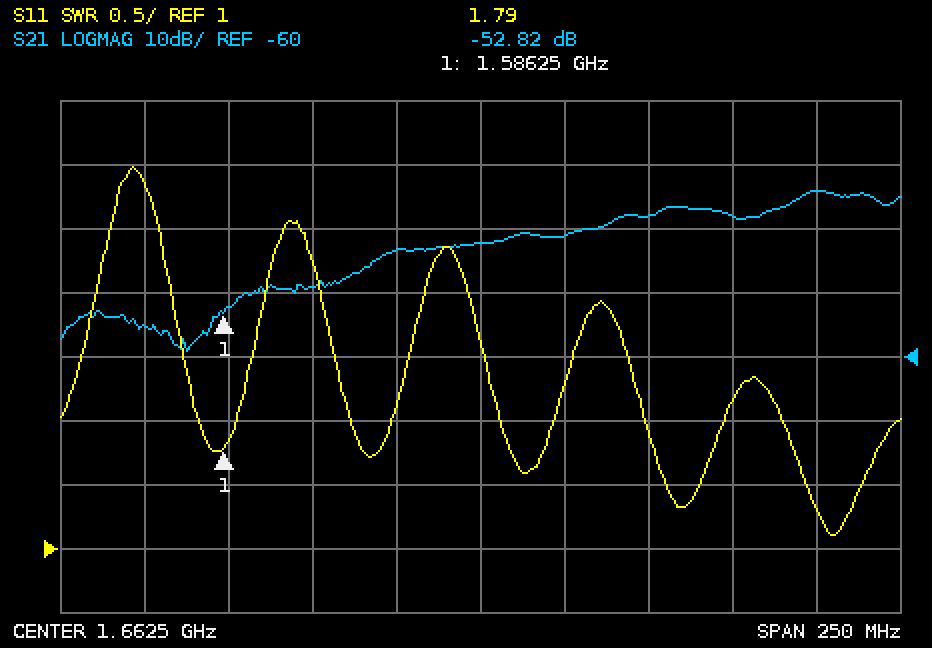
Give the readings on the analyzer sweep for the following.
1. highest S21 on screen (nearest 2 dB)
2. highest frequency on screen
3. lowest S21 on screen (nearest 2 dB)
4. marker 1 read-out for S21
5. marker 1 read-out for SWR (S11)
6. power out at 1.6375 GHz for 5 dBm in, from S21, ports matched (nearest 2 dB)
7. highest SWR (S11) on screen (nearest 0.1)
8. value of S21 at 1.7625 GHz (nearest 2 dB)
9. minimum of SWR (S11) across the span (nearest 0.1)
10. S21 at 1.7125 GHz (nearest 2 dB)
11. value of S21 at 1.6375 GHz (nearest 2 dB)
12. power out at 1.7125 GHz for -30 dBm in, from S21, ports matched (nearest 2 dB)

-34 dB
1.7875 GHz
-60 dB
-52.82 dB
1.79
-38 dBm
4.0
-34 dB
1.1
-38 dB
-44 dB
-68 dBm
